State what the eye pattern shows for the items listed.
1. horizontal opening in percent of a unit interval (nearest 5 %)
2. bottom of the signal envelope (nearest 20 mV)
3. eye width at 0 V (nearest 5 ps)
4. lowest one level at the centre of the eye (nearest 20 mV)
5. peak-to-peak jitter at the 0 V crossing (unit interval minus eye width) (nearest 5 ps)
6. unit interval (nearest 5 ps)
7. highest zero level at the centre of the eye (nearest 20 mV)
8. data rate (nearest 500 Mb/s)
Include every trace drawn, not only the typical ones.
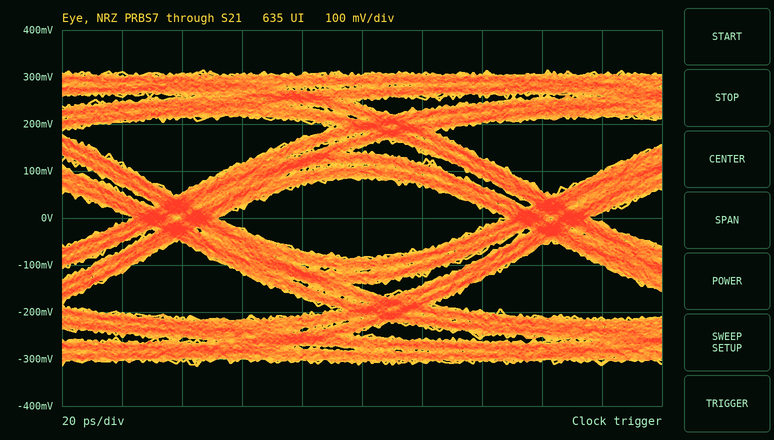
75 %
-320 mV
95 ps
80 mV
30 ps
125 ps
-80 mV
8.0 Gb/s
